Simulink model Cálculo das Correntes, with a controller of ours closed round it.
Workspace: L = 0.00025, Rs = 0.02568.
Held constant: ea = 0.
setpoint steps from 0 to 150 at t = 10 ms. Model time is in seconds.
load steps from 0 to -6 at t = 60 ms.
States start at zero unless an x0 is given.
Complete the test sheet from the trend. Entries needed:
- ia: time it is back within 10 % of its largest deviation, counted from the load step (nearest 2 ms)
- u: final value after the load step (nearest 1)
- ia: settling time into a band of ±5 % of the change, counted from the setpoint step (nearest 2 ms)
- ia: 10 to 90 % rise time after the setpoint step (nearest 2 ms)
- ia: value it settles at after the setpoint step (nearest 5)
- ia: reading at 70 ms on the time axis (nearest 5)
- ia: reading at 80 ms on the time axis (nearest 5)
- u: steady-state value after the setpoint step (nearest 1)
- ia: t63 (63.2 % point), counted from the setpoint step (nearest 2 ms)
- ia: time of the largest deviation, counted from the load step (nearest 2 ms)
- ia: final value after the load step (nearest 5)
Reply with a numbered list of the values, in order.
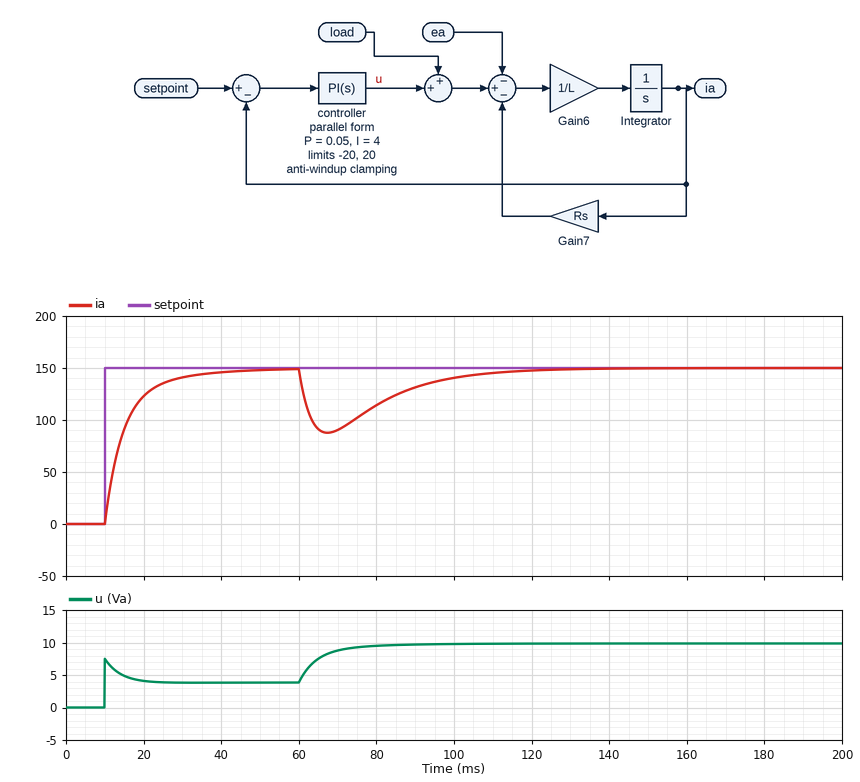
1. 46 ms
2. 10
3. 22 ms
4. 14 ms
5. 150
6. 90
7. 115
8. 4
9. 6 ms
10. 8 ms
11. 150
